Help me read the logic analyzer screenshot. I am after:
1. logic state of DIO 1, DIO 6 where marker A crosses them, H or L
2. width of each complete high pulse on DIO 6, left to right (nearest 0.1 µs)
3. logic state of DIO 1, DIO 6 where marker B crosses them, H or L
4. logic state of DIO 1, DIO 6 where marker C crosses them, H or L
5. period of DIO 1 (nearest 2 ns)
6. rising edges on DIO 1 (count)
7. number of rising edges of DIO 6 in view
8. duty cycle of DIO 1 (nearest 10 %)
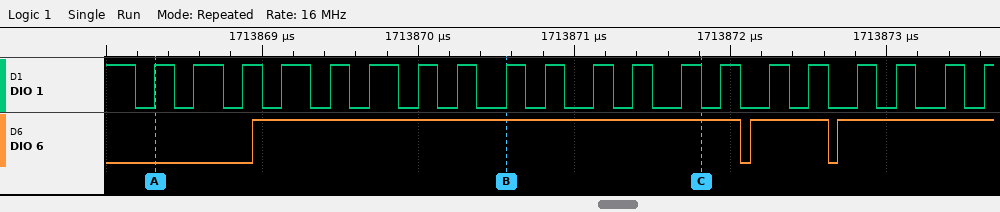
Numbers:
DIO 1=H, DIO 6=L
3.1 µs, 0.5 µs
DIO 1=H, DIO 6=H
DIO 1=L, DIO 6=H
280 ns
20
3
50 %
